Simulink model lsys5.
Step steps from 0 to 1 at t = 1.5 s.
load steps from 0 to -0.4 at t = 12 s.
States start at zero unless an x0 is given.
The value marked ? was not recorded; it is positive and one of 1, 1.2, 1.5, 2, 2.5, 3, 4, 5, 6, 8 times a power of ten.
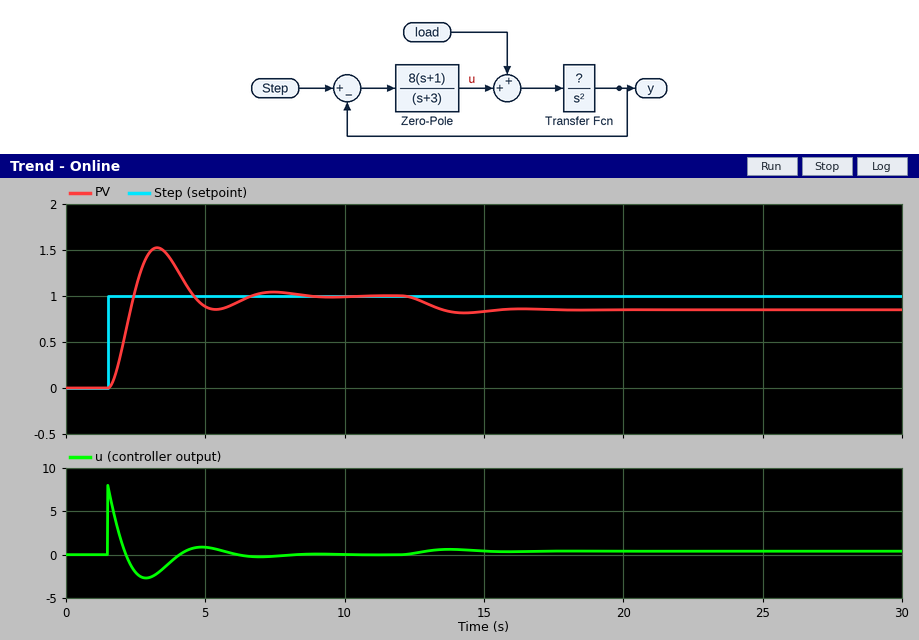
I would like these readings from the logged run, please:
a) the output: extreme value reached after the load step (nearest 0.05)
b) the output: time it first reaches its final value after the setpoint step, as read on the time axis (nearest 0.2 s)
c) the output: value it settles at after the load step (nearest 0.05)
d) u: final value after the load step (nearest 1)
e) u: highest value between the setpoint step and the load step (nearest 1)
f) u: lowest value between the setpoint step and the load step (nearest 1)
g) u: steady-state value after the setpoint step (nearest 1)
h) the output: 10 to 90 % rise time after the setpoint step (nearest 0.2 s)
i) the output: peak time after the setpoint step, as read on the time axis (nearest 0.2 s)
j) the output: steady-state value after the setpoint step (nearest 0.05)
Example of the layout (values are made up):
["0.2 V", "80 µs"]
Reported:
["0.80", "2.4 s", "0.85", "0", "8", "-3", "0", "0.6 s", "3.2 s", "1.00"]
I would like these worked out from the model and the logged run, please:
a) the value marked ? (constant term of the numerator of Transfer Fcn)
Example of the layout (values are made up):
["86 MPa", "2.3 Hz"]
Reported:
["0.6"]
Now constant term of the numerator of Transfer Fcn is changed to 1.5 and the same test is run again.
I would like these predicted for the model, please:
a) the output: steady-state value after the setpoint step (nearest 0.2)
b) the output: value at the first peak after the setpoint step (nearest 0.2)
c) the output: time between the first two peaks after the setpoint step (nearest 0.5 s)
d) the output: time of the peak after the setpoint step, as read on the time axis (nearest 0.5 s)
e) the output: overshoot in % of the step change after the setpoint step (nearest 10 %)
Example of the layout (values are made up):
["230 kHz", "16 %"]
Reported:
["1.0", "1.6", "2.0 s", "2.5 s", "60 %"]
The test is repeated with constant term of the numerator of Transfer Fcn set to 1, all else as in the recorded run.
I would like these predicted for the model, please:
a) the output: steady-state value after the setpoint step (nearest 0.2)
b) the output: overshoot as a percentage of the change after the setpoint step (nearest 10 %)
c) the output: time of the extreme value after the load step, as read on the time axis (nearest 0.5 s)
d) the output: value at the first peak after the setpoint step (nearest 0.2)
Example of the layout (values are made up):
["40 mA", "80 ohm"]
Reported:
["1.0", "50 %", "13.5 s", "1.6"]
